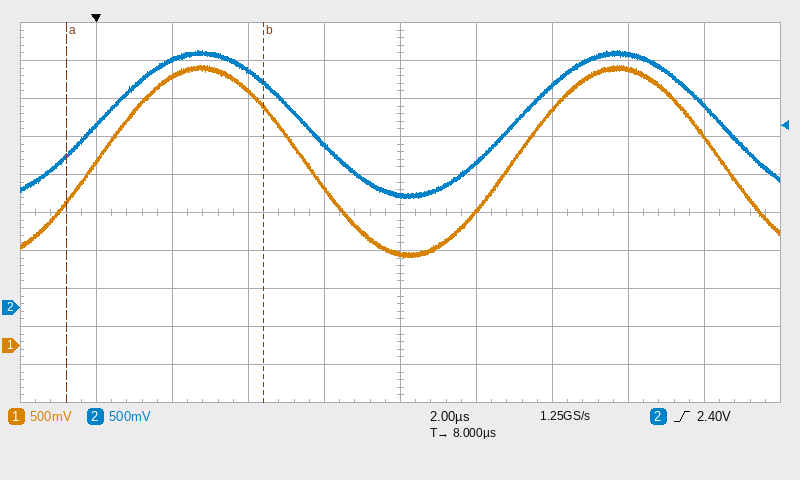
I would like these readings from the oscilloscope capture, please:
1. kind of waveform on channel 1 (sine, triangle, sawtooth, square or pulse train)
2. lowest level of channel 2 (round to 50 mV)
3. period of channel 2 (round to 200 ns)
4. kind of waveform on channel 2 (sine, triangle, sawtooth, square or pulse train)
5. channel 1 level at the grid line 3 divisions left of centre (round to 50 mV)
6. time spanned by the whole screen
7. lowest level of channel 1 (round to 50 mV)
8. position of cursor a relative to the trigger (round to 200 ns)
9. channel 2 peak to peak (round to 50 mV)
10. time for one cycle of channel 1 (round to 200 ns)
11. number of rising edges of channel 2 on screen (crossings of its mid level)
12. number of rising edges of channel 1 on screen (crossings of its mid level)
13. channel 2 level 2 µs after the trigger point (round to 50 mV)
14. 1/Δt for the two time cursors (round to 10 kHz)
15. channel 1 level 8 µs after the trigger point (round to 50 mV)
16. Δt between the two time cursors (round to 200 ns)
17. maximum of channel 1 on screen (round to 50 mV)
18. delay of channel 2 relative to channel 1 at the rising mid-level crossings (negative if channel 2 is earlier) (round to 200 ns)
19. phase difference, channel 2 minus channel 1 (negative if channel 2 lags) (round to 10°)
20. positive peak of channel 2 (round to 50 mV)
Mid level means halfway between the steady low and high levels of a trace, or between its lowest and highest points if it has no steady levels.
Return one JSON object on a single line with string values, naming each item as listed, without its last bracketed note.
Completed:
{"kind of waveform on channel 1": "sine", "lowest level of channel 2": "1.45 V", "period of channel 2": "11.0 µs", "kind of waveform on channel 2": "sine", "channel 1 level at the grid line 3 divisions left of centre": "3.55 V", "time spanned by the whole screen": "20 µs", "lowest level of channel 1": "1.15 V", "position of cursor a relative to the trigger": "-800 ns", "channel 2 peak to peak": "1.95 V", "time for one cycle of channel 1": "11.0 µs", "number of rising edges of channel 2 on screen": "2", "number of rising edges of channel 1 on screen": "2", "channel 2 level 2 µs after the trigger point": "3.25 V", "1/Δt for the two time cursors": "190 kHz", "channel 1 level 8 µs after the trigger point": "1.20 V", "Δt between the two time cursors": "5.2 µs", "maximum of channel 1 on screen": "3.70 V", "delay of channel 2 relative to channel 1 at the rising mid-level crossings (negative if channel 2 is earlier)": "0.0 µs", "phase difference, channel 2 minus channel 1 (negative if channel 2 lags)": "0°", "positive peak of channel 2": "3.40 V"}
